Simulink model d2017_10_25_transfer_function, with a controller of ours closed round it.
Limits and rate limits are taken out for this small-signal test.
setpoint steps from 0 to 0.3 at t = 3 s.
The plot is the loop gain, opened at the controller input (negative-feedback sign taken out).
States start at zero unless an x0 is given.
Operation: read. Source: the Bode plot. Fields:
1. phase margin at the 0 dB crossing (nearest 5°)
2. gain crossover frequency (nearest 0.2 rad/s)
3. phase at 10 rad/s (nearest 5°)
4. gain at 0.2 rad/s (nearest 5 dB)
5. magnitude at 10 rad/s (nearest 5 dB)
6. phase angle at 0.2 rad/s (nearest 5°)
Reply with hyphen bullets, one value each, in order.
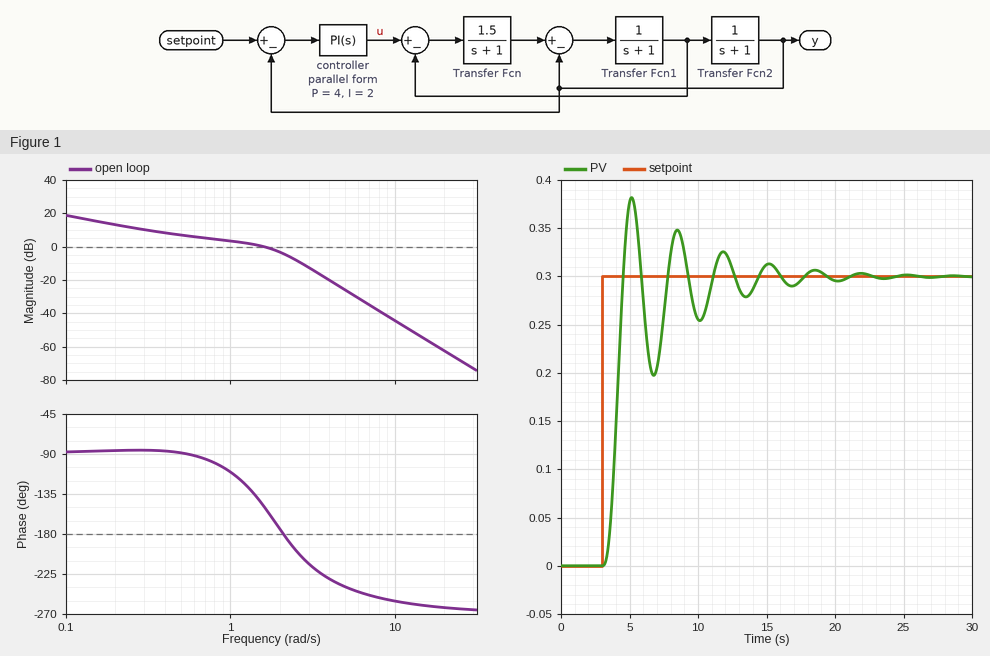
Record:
- 30°
- 1.6 rad/s
- -255°
- 15 dB
- -45 dB
- -85°
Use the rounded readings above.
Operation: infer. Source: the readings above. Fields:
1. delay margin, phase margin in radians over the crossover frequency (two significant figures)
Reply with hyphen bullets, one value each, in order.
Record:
- 0.33 s
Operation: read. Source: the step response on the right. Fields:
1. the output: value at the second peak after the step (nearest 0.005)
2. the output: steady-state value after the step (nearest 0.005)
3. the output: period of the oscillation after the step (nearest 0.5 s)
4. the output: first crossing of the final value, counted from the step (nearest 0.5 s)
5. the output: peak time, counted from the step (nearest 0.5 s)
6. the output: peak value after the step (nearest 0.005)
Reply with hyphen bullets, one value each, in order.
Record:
- 0.350
- 0.300
- 3.5 s
- 1.5 s
- 2.0 s
- 0.380
